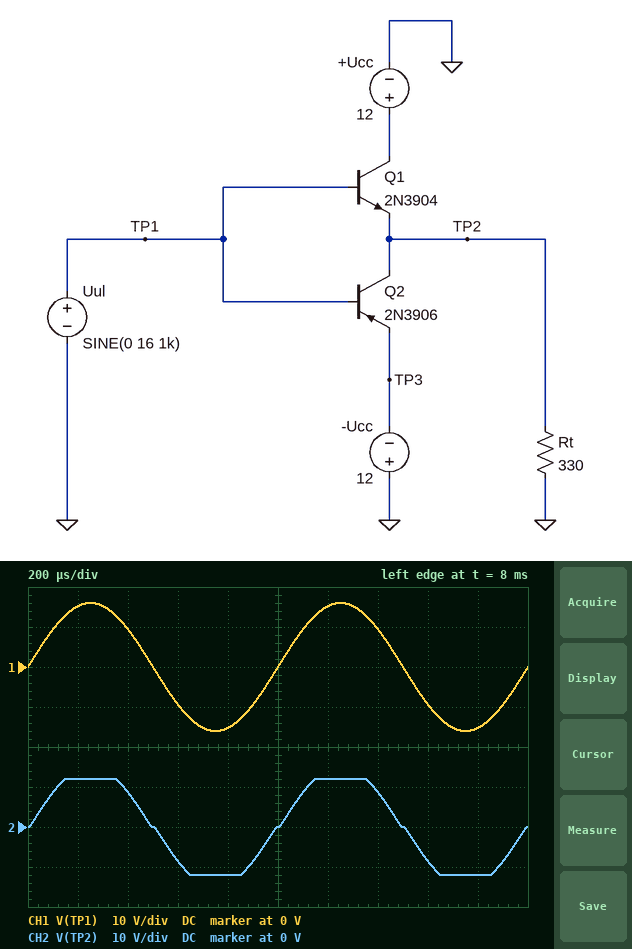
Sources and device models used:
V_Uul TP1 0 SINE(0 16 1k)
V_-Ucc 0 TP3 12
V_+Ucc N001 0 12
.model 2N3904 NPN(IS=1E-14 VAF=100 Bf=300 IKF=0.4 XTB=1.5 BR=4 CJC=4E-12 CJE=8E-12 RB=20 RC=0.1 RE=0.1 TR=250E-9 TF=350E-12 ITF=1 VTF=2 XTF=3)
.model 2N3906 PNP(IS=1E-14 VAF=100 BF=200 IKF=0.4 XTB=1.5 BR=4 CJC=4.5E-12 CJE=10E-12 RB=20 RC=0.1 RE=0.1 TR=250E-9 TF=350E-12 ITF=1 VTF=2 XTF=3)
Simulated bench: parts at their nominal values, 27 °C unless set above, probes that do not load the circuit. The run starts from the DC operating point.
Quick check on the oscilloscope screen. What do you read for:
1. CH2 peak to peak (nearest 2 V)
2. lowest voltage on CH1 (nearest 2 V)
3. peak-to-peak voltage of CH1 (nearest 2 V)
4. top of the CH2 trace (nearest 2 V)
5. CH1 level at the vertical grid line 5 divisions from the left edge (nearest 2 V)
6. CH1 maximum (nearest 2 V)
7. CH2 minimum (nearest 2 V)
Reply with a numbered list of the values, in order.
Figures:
1. 24 V
2. -16 V
3. 32 V
4. 12 V
5. 0 V
6. 16 V
7. -12 V
